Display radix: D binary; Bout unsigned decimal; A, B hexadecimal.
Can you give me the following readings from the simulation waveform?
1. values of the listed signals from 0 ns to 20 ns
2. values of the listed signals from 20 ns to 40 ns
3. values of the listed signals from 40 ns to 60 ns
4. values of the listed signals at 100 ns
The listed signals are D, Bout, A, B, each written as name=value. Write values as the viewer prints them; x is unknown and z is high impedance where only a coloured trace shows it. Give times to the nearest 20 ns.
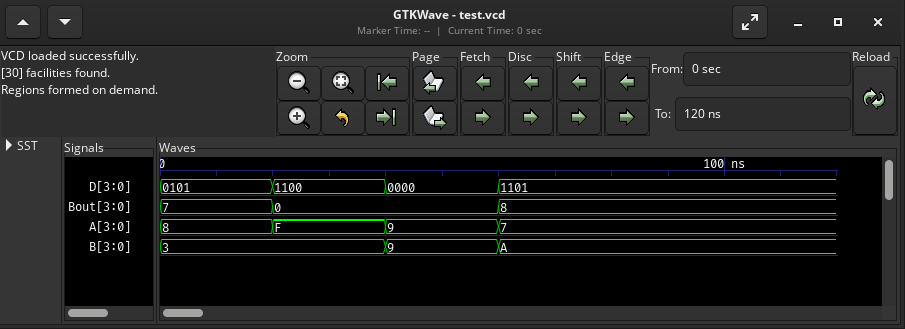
D=0101, Bout=7, A=8, B=3
D=1100, Bout=0, A=F, B=3
D=0000, Bout=0, A=9, B=9
D=1101, Bout=8, A=7, B=A
